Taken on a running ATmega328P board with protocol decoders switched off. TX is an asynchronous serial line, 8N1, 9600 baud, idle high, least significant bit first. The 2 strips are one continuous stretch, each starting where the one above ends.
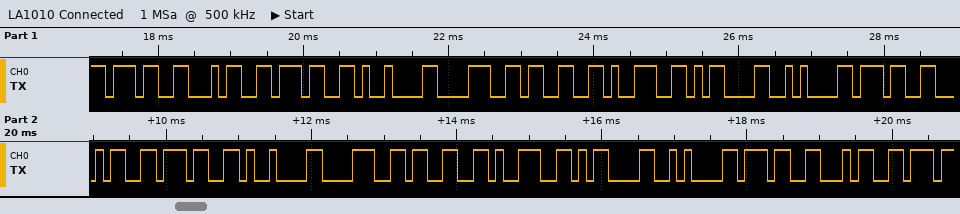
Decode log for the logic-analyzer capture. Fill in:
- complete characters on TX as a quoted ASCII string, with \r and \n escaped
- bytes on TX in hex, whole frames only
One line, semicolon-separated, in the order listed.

"747\t839\r\n747\t839\r\n74"; 0x37 0x34 0x37 0x09 0x38 0x33 0x39 0x0D 0x0A 0x37 0x34 0x37 0x09 0x38 0x33 0x39 0x0D 0x0A 0x37 0x34
